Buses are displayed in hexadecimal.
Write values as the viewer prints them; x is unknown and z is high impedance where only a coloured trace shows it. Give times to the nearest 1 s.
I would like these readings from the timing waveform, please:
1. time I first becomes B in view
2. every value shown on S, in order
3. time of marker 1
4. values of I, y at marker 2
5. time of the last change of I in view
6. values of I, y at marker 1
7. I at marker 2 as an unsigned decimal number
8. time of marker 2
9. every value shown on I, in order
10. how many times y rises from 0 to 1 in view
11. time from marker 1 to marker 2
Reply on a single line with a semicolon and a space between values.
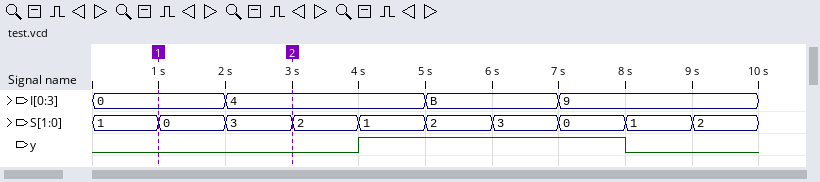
5 s; 1, 0, 3, 2, 1, 2, 3, 0, 1, 2; 1 s; I=4, y=0; 7 s; I=0, y=0; 4; 3 s; 0, 4, B, 9; 1; 2 s
